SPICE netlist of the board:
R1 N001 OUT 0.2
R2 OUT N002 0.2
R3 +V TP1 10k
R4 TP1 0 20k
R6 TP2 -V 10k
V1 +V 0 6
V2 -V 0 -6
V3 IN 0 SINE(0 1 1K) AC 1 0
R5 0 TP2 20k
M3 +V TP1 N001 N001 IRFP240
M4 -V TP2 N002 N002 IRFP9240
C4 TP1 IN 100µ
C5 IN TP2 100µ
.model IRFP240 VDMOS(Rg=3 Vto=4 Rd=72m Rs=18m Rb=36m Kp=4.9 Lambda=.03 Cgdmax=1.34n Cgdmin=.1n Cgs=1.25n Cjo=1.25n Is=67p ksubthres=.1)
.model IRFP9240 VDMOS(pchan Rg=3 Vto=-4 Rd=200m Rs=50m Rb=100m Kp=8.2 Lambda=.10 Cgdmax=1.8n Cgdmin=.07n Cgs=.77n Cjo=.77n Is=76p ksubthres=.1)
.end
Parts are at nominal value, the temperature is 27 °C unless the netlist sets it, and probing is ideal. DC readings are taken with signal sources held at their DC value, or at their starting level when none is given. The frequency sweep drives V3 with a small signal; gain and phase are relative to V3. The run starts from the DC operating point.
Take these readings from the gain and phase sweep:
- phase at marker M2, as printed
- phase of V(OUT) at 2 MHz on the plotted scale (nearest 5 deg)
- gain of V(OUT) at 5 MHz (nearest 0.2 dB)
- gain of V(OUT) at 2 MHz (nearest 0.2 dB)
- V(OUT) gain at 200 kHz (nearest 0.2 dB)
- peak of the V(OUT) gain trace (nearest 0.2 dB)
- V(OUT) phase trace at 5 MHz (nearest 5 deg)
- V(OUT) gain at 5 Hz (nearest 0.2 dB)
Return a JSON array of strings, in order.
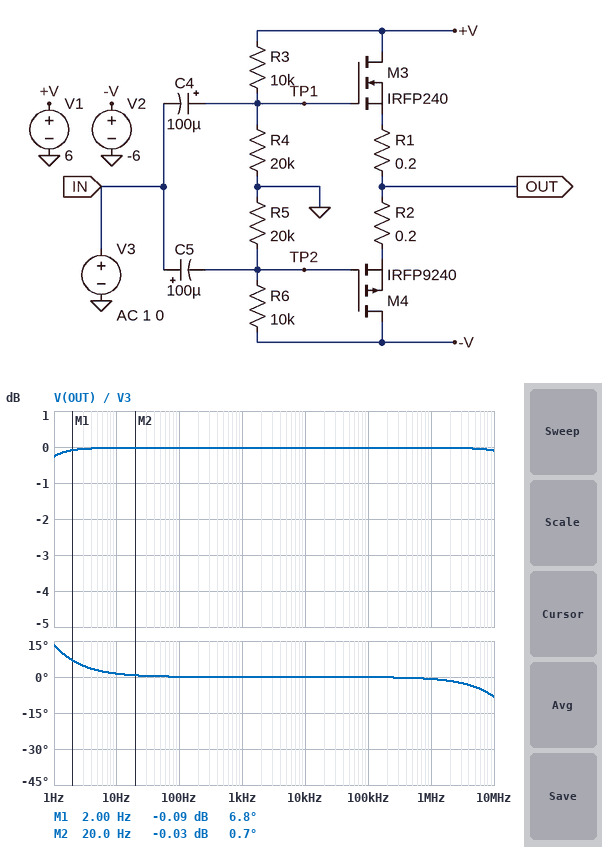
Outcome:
["0.7 deg", "0 deg", "0 dB", "0 dB", "0 dB", "0 dB", "-5 deg", "0 dB"]
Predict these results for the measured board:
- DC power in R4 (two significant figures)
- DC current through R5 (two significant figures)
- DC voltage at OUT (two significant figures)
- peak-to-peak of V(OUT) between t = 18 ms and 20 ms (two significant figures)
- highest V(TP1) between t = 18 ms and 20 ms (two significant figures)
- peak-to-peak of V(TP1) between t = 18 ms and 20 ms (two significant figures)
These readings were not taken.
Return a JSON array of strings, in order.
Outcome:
["800 µW", "200 µA", "-28 mV", "2.0 V", "5.0 V", "2.0 V"]
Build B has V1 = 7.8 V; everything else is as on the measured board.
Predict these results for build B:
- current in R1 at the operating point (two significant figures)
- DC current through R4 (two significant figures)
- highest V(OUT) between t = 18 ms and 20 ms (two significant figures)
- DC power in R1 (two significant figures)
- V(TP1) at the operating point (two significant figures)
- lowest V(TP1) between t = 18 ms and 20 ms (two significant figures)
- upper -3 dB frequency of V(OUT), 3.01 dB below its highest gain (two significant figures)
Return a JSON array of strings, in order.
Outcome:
["760 mA", "260 µA", "1.5 V", "120 mW", "5.2 V", "4.2 V", "150 MHz"]
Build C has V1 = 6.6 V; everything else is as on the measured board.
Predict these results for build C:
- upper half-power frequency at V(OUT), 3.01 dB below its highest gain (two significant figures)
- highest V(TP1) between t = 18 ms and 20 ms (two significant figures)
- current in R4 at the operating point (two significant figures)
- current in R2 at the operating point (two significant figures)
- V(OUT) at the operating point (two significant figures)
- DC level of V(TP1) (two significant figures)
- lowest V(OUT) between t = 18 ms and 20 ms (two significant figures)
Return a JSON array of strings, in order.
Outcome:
["120 MHz", "5.4 V", "220 µA", "140 mA", "160 mV", "4.4 V", "-840 mV"]
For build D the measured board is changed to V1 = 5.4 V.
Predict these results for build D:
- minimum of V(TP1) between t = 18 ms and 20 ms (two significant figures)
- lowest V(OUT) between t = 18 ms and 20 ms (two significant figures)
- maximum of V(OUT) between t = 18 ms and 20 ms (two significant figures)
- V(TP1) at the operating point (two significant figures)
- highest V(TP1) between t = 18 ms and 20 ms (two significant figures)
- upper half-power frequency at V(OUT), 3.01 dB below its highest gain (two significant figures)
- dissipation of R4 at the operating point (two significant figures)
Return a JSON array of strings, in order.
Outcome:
["2.6 V", "-1.2 V", "780 mV", "3.6 V", "4.6 V", "28 MHz", "650 µW"]
